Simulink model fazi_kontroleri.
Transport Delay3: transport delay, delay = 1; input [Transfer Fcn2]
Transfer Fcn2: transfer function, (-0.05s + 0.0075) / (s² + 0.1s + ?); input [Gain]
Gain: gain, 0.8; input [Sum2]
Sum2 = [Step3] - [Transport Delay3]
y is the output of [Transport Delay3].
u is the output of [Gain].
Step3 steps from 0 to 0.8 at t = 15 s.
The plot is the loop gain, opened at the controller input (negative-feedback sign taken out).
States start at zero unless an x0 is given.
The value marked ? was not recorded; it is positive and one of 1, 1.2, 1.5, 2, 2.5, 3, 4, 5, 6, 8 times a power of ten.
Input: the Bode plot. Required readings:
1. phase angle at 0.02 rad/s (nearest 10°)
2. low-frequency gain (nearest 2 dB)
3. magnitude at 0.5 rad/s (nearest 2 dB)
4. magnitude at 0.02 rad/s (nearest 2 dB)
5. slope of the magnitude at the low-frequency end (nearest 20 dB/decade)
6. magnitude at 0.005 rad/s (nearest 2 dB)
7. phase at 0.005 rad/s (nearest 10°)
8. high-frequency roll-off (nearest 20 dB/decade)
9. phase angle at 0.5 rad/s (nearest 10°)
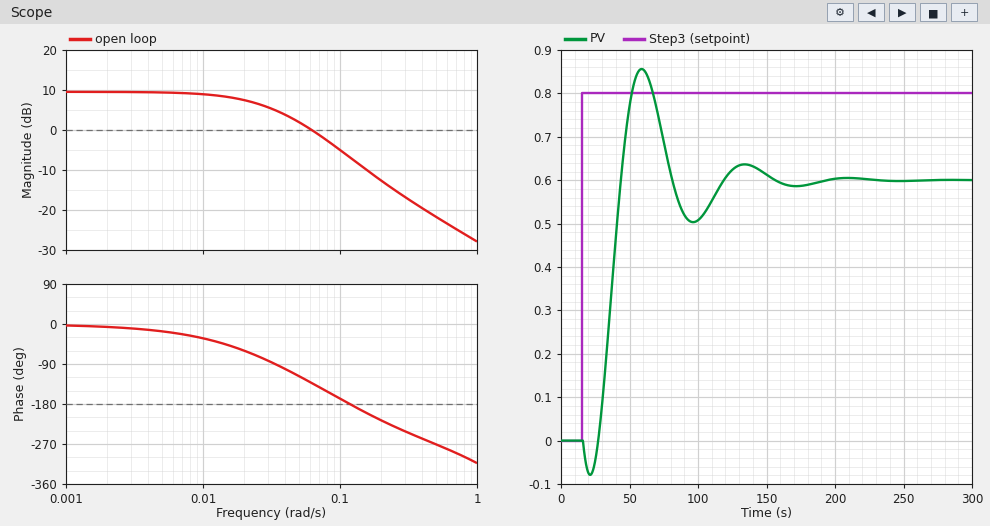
-60°
10 dB
-22 dB
8 dB
0 dB/decade
10 dB
-20°
-20 dB/decade
-270°
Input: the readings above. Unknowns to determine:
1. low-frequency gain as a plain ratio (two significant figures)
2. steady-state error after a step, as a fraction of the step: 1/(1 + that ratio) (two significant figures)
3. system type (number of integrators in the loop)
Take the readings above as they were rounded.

3.2
0.24
0
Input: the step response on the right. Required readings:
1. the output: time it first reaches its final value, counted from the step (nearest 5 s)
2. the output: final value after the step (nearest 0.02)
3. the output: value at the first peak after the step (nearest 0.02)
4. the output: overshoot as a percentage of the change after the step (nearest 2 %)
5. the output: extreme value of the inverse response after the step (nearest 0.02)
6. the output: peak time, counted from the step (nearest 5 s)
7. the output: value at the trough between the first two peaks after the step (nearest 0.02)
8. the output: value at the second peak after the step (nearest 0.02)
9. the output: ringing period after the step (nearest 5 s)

30 s
0.60
0.86
42 %
-0.08
45 s
0.50
0.64
75 s
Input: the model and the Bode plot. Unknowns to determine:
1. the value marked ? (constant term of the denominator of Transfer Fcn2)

0.002
